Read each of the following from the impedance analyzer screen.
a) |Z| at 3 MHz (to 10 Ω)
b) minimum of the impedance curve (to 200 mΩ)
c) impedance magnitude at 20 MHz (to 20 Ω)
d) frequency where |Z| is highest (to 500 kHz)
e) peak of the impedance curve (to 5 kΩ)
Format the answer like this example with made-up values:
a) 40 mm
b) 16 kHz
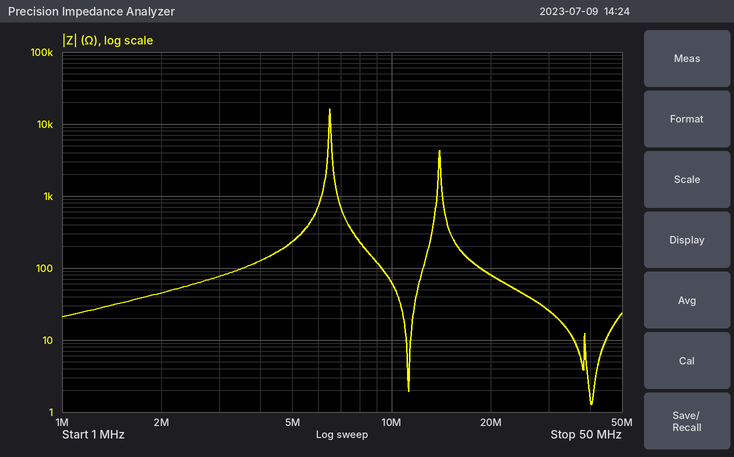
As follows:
a) 80 Ω
b) 1.2 Ω
c) 80 Ω
d) 6.5 MHz
e) 15 kΩ
